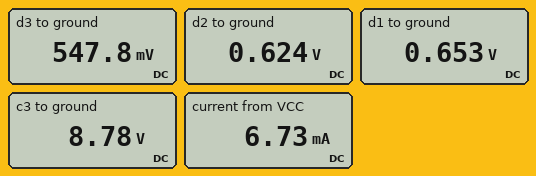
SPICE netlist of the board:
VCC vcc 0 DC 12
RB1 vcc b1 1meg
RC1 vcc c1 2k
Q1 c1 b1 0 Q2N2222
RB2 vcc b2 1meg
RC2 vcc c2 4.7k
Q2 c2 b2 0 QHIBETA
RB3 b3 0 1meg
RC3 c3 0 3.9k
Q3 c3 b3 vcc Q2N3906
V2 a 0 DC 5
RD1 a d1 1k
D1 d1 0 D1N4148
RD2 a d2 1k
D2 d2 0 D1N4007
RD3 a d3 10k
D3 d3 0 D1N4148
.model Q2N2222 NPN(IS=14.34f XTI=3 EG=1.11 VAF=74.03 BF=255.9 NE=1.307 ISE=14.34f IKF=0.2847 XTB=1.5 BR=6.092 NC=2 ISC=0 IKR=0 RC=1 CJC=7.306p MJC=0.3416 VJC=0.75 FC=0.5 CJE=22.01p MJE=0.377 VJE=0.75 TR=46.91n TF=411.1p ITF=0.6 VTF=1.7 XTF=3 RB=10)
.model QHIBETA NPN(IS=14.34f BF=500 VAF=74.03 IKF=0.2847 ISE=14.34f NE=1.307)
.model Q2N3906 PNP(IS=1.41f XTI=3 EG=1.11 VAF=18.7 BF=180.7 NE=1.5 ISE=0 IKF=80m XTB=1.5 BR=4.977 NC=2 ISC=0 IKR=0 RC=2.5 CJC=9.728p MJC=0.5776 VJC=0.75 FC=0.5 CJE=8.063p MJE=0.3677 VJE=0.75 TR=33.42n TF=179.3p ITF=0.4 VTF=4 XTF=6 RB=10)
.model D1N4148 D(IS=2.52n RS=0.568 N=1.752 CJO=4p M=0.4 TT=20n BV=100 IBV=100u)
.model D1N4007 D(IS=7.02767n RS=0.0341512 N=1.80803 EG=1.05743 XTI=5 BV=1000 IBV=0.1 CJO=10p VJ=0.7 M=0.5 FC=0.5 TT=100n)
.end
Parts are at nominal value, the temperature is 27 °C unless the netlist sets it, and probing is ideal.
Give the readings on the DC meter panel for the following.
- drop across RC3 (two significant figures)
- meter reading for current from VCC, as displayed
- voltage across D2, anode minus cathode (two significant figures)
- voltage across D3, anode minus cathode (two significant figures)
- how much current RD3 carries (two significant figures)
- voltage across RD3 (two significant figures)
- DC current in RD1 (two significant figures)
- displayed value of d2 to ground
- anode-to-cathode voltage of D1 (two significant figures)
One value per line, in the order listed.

8.8 V
6.73 mA
620 mV
550 mV
450 µA
4.5 V
4.3 mA
0.624 V
650 mV
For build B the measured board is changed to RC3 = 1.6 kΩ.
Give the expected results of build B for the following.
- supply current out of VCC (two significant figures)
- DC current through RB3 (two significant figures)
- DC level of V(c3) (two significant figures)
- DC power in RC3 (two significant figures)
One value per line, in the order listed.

7.2 mA
11 µA
4.4 V
12 mW
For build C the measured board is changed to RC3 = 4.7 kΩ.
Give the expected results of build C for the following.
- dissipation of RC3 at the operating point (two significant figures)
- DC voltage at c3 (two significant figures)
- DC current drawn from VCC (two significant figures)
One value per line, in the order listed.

21 mW
10 V
6.6 mA
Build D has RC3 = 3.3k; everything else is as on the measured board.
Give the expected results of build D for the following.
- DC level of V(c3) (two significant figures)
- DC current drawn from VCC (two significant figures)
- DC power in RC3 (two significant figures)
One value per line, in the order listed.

7.8 V
6.8 mA
18 mW
